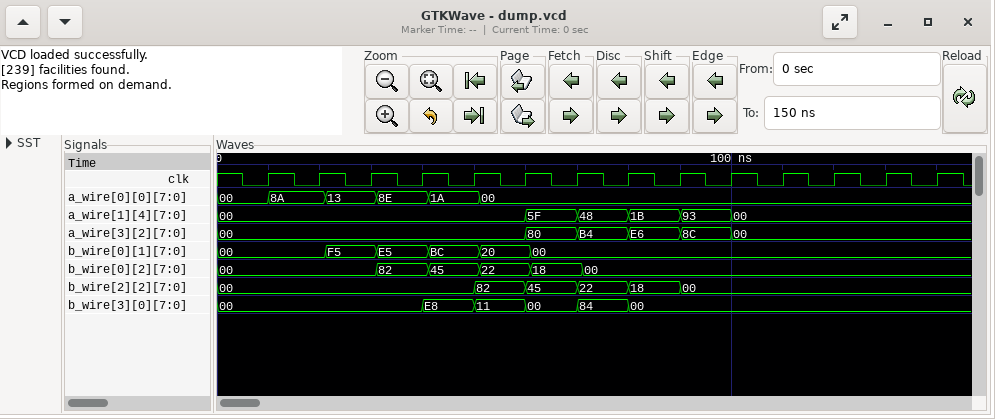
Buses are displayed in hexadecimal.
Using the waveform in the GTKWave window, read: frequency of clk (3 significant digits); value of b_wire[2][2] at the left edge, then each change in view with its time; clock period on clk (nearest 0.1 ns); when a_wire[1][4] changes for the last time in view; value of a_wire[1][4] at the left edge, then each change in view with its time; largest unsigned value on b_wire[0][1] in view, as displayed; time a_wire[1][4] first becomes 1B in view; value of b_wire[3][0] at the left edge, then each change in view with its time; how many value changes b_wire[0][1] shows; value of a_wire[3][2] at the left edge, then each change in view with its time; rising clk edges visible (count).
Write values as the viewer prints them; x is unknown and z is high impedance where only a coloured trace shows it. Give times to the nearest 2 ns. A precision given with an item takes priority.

100 MHz
00, 82 at 50 ns, 45 at 60 ns, 22 at 70 ns, 18 at 80 ns, 00 at 90 ns
10 ns
100 ns
00, 5F at 60 ns, 48 at 70 ns, 1B at 80 ns, 93 at 90 ns, 00 at 100 ns
F5
80 ns
00, E8 at 40 ns, 11 at 50 ns, 00 at 60 ns, 84 at 70 ns, 00 at 80 ns
5
00, 80 at 60 ns, B4 at 70 ns, E6 at 80 ns, 8C at 90 ns, 00 at 100 ns
14
